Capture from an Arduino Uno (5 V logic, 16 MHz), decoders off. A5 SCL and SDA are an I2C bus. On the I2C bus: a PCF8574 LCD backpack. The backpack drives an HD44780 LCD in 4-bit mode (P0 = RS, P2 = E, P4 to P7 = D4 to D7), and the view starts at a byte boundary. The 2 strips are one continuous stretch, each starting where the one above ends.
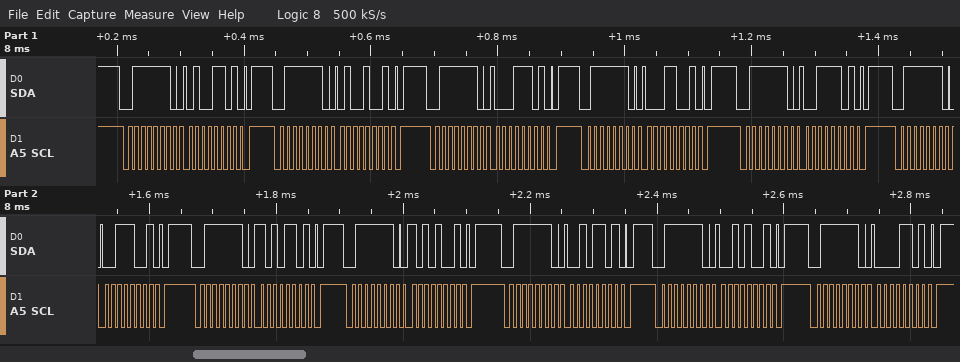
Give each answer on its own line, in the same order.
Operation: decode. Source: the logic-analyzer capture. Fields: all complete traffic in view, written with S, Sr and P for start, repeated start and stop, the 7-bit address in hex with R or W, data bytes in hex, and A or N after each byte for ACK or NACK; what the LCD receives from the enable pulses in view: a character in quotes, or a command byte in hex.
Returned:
S 3FW A 4D A P S 3FW A 49 A P S 3FW A 1D A P S 3FW A 19 A P S 3FW A 3D A P S 3FW A 39 A P S 3FW A AD A P S 3FW A A9 A P S 3FW A 2D A P S 3FW A 29 A P S 3FW A 0D A P
'A' ':'
